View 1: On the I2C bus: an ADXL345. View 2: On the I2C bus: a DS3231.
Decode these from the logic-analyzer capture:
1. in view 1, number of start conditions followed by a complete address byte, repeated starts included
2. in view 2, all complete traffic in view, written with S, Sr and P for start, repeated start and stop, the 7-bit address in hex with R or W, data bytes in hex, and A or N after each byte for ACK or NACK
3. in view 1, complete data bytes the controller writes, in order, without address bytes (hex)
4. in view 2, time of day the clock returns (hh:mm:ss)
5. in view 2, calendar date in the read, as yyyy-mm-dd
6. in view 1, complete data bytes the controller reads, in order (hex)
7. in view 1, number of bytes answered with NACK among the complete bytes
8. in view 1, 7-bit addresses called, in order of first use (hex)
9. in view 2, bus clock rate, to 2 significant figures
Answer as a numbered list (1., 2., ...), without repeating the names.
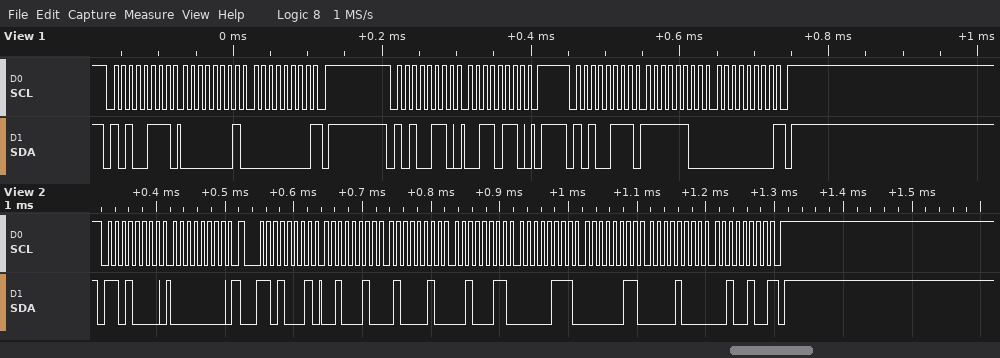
1. 3
2. S 68W A 00 A Sr 68R A 22 A 42 A 23 A 07 A 03 A 08 A 24 N P
3. 36
4. 23:42:22
5. 2024-08-03
6. 01 00 FC 00
7. 2
8. 0x53
9. 100 kHz
